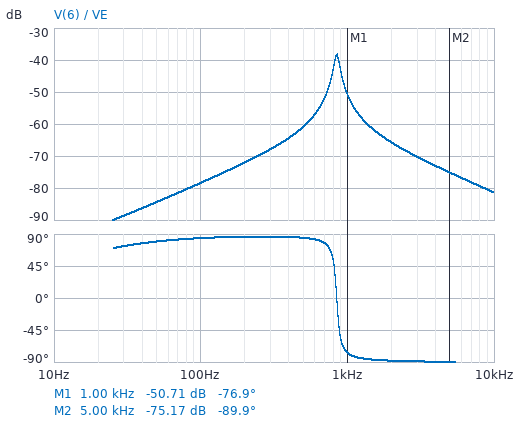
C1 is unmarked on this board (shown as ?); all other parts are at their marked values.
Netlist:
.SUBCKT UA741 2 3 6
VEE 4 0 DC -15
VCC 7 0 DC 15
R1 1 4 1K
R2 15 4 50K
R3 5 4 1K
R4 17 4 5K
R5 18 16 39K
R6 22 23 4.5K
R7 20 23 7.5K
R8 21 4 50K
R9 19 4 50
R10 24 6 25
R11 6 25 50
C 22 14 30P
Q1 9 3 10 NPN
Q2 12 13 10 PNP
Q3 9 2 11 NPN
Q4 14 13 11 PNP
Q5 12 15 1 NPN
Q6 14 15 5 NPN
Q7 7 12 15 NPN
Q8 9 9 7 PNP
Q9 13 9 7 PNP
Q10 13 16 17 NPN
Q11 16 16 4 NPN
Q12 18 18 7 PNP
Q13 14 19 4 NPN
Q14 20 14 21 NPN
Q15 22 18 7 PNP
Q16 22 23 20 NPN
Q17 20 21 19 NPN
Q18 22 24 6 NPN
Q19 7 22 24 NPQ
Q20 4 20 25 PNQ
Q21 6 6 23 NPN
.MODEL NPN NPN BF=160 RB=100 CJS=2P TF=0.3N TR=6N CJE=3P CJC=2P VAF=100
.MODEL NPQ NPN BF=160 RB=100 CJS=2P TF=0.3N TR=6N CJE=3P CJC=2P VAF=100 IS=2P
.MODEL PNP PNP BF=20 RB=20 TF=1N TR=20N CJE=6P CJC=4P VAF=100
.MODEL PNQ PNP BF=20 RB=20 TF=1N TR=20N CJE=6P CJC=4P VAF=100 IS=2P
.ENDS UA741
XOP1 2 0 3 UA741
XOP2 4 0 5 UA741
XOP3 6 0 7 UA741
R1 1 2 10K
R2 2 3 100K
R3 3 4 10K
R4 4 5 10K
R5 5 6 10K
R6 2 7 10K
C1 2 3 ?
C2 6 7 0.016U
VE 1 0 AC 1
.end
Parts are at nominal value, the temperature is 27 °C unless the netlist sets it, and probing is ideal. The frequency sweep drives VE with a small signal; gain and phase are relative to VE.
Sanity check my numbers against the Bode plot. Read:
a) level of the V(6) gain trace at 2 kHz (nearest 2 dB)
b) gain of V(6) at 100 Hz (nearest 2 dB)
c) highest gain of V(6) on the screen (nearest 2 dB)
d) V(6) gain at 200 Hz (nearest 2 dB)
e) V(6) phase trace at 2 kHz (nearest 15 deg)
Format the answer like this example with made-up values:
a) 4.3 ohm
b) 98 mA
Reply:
a) -66 dB
b) -78 dB
c) -38 dB
d) -72 dB
e) -90 deg
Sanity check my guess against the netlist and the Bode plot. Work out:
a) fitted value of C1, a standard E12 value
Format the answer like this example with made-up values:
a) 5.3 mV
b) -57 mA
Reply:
a) 22 nF
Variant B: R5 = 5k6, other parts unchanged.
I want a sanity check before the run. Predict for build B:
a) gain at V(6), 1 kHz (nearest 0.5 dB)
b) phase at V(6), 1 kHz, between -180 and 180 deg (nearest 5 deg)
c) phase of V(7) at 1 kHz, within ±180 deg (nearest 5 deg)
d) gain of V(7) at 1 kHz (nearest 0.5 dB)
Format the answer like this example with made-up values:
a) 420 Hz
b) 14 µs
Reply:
a) -45.5 dB
b) 75 deg
c) 165 deg
d) 13.0 dB
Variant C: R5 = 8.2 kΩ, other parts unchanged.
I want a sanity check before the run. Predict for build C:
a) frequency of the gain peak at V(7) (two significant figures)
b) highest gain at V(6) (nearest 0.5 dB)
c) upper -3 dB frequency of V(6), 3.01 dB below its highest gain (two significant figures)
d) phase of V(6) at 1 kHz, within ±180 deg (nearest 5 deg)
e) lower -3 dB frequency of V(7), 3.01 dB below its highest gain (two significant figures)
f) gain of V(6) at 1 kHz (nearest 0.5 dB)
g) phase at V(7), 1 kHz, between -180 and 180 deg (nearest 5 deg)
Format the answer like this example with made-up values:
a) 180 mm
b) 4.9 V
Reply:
a) 930 Hz
b) -36.5 dB
c) 970 Hz
d) -60 deg
e) 900 Hz
f) -43.0 dB
g) 30 deg
